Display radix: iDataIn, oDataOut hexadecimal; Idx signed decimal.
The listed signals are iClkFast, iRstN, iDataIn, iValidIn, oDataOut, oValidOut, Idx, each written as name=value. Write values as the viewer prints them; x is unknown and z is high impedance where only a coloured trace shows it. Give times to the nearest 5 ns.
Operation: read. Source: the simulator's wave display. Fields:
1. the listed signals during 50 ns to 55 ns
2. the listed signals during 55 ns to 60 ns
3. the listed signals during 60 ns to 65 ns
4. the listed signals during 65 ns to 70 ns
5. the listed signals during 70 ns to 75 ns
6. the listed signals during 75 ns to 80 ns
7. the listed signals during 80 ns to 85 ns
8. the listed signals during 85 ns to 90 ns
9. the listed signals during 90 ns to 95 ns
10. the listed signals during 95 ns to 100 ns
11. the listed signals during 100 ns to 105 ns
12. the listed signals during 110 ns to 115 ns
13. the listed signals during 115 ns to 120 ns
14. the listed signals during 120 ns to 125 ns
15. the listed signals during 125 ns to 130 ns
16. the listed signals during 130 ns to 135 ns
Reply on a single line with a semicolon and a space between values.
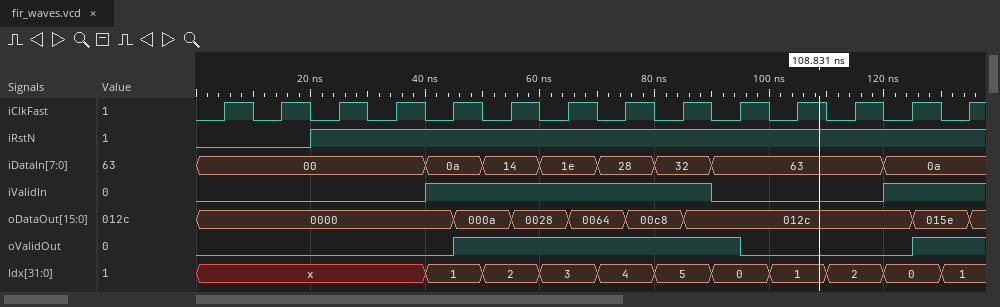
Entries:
iClkFast=0, iRstN=1, iDataIn=14, iValidIn=1, oDataOut=000a, oValidOut=1, Idx=2; iClkFast=1, iRstN=1, iDataIn=14, iValidIn=1, oDataOut=0028, oValidOut=1, Idx=2; iClkFast=0, iRstN=1, iDataIn=1e, iValidIn=1, oDataOut=0028, oValidOut=1, Idx=3; iClkFast=1, iRstN=1, iDataIn=1e, iValidIn=1, oDataOut=0064, oValidOut=1, Idx=3; iClkFast=0, iRstN=1, iDataIn=28, iValidIn=1, oDataOut=0064, oValidOut=1, Idx=4; iClkFast=1, iRstN=1, iDataIn=28, iValidIn=1, oDataOut=00c8, oValidOut=1, Idx=4; iClkFast=0, iRstN=1, iDataIn=32, iValidIn=1, oDataOut=00c8, oValidOut=1, Idx=5; iClkFast=1, iRstN=1, iDataIn=32, iValidIn=1, oDataOut=012c, oValidOut=1, Idx=5; iClkFast=0, iRstN=1, iDataIn=63, iValidIn=0, oDataOut=012c, oValidOut=1, Idx=0; iClkFast=1, iRstN=1, iDataIn=63, iValidIn=0, oDataOut=012c, oValidOut=0, Idx=0; iClkFast=0, iRstN=1, iDataIn=63, iValidIn=0, oDataOut=012c, oValidOut=0, Idx=1; iClkFast=0, iRstN=1, iDataIn=63, iValidIn=0, oDataOut=012c, oValidOut=0, Idx=2; iClkFast=1, iRstN=1, iDataIn=63, iValidIn=0, oDataOut=012c, oValidOut=0, Idx=2; iClkFast=0, iRstN=1, iDataIn=0a, iValidIn=1, oDataOut=012c, oValidOut=0, Idx=0; iClkFast=1, iRstN=1, iDataIn=0a, iValidIn=1, oDataOut=015e, oValidOut=1, Idx=0; iClkFast=0, iRstN=1, iDataIn=0a, iValidIn=1, oDataOut=015e, oValidOut=1, Idx=1
